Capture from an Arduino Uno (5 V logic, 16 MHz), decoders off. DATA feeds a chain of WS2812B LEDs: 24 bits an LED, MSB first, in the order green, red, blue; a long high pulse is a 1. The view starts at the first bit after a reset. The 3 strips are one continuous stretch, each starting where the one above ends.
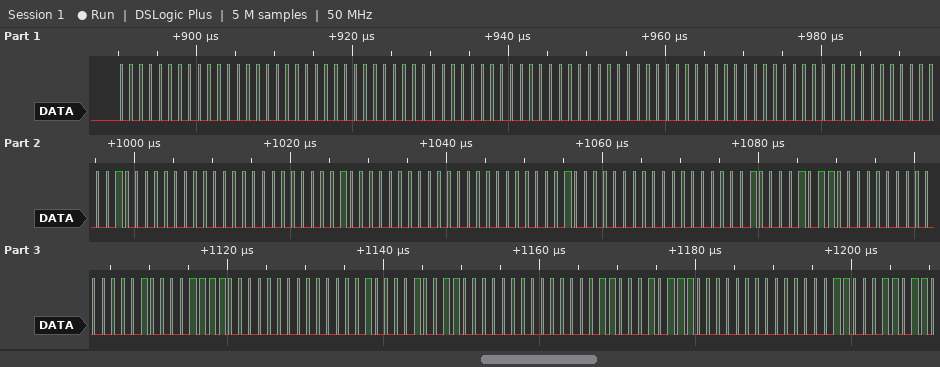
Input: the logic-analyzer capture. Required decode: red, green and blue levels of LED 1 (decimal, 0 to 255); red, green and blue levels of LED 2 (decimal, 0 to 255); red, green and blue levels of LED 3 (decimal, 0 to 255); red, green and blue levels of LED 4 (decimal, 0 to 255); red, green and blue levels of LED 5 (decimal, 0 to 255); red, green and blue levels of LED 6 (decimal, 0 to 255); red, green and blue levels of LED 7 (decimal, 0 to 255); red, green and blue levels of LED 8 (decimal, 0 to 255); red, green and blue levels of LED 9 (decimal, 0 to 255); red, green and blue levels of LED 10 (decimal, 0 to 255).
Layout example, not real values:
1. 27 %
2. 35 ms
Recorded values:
1. 0, 0, 0
2. 0, 0, 0
3. 0, 0, 0
4. 2, 0, 0
5. 4, 0, 0
6. 8, 0, 0
7. 11, 1, 0
8. 15, 1, 0
9. 19, 2, 0
10. 23, 3, 0
